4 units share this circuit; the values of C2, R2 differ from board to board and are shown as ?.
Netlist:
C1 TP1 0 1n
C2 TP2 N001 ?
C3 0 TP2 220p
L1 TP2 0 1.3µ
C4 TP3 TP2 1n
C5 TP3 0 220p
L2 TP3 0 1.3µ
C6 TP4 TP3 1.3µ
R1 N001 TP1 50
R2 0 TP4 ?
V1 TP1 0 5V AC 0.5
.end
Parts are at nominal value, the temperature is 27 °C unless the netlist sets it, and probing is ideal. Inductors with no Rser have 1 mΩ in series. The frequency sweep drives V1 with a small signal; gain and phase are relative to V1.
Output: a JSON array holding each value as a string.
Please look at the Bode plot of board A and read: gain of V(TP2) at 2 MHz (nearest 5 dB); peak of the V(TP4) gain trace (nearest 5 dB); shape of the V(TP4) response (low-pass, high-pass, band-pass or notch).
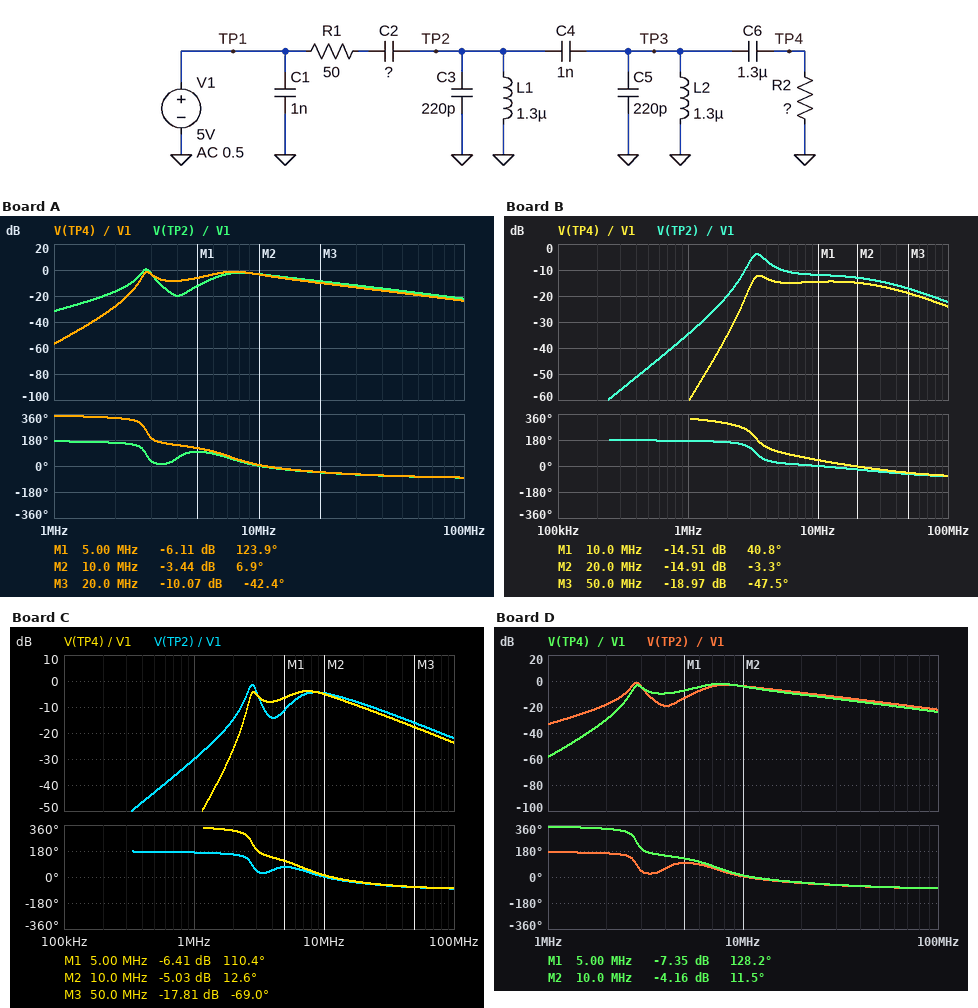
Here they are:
["-15 dB", "0 dB", "band-pass"]
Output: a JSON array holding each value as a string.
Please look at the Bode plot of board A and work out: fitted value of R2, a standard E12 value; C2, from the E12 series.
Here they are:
["150 Ω", "470 pF"]
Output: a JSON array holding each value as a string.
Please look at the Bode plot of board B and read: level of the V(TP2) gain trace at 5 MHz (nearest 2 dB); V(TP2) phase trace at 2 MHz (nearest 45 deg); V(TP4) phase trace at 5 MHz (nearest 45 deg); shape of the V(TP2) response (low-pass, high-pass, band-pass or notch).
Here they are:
["-10 dB", "180 deg", "90 deg", "band-pass"]
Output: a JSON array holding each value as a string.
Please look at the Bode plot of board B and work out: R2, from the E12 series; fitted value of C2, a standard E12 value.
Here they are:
["18 Ω", "330 pF"]
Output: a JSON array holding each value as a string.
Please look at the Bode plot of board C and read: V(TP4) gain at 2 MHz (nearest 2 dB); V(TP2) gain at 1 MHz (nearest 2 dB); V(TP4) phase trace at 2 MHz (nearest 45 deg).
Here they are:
["-26 dB", "-30 dB", "315 deg"]
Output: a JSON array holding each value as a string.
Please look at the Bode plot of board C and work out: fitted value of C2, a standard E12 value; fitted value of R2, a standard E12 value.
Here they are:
["560 pF", "82 Ω"]
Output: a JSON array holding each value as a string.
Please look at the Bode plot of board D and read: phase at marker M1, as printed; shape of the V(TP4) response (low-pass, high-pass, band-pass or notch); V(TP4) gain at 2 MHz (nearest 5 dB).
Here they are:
["128.2 deg", "band-pass", "-30 dB"]
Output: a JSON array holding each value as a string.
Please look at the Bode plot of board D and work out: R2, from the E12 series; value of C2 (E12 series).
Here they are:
["120 Ω", "390 pF"]
